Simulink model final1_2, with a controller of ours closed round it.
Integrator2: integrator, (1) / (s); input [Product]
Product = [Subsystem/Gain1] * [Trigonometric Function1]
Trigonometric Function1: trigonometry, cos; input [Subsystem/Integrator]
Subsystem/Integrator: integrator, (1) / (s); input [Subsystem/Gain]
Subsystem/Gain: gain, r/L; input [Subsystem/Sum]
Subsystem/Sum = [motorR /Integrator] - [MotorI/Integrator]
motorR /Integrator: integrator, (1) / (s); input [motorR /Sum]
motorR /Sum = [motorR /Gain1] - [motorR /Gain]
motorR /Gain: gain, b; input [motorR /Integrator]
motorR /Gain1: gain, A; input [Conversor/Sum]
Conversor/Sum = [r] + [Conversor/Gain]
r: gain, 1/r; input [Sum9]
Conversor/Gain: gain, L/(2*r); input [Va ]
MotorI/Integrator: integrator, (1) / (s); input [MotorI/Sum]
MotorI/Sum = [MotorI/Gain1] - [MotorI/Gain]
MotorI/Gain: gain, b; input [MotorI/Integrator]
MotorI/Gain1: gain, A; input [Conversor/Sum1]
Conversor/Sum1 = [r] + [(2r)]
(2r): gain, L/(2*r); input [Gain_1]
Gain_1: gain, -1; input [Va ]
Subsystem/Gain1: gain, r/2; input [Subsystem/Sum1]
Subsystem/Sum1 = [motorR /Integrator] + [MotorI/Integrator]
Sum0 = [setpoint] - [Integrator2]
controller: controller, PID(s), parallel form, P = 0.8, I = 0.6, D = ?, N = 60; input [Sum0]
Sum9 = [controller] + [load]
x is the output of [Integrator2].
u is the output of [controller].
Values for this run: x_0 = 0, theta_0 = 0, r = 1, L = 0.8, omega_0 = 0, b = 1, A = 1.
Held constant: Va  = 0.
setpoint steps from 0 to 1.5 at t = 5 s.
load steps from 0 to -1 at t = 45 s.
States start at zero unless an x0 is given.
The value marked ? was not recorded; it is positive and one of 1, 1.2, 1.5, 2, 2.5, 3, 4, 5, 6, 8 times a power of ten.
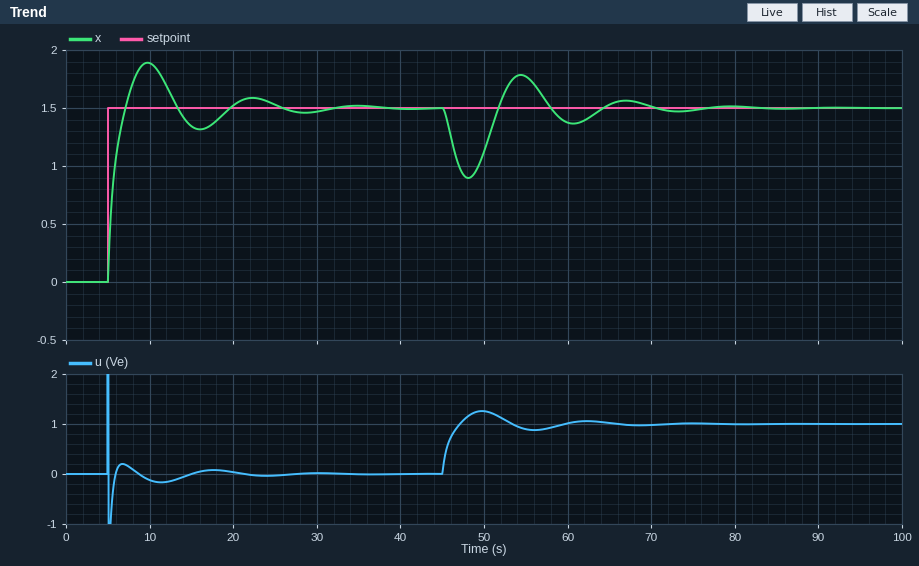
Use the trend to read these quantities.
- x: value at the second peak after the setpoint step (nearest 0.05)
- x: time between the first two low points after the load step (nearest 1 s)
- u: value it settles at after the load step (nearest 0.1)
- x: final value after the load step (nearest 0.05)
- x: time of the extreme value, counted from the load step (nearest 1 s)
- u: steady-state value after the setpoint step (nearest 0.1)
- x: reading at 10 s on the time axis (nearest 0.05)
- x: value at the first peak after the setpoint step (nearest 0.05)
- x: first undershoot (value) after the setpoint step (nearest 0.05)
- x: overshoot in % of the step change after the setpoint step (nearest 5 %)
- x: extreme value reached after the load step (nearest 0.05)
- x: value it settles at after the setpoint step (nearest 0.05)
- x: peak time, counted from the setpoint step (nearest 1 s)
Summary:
1.60
13 s
1.0
1.50
3 s
0.0
1.90
1.90
1.30
25 %
0.90
1.50
5 s
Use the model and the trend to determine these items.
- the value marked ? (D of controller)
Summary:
1.5
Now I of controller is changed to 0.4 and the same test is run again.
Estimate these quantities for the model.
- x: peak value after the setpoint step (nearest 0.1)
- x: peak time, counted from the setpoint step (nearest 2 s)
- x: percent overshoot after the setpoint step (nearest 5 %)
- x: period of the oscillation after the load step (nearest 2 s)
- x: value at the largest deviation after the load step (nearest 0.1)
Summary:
1.8
6 s
20 %
16 s
0.8
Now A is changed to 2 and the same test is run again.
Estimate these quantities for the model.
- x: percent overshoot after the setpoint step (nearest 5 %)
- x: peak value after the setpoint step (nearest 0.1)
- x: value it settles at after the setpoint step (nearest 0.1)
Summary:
15 %
1.7
1.5
